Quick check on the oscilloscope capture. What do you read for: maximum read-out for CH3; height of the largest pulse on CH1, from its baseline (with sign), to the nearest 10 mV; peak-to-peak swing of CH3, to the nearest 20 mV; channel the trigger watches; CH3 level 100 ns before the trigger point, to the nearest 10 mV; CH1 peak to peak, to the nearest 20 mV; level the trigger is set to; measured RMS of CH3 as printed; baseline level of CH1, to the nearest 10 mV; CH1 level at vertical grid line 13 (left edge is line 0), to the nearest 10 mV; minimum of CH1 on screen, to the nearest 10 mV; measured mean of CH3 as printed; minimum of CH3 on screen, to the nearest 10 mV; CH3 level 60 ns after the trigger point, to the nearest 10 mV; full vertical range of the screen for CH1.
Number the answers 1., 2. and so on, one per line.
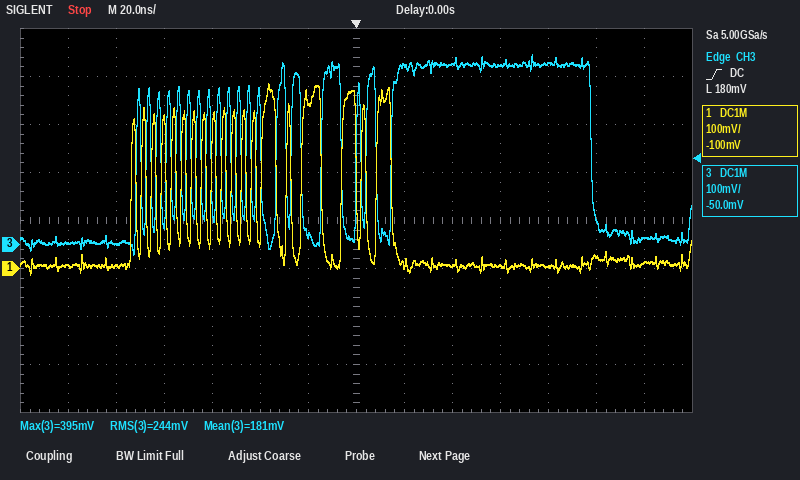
1. 395 mV
2. +380 mV
3. 420 mV
4. CH3
5. 0 mV
6. 400 mV
7. 180 mV
8. 244 mV
9. 10 mV
10. 10 mV
11. -10 mV
12. 181 mV
13. -20 mV
14. 370 mV
15. 800 mV
